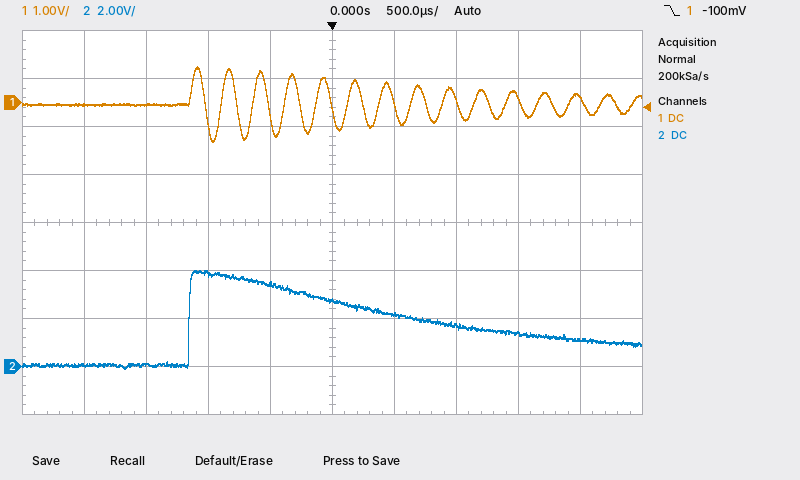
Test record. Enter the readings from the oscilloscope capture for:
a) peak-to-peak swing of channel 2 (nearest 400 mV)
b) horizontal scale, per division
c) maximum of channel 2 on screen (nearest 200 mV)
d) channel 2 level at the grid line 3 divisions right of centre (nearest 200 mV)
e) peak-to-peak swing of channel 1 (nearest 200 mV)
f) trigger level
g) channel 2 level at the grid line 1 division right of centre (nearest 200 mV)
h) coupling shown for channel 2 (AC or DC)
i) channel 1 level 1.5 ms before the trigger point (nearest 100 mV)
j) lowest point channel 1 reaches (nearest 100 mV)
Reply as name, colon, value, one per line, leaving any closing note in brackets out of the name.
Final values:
peak-to-peak swing of channel 2: 4.0 V
horizontal scale, per division: 500 µs
maximum of channel 2 on screen: 4.0 V
channel 2 level at the grid line 3 divisions right of centre: 1.4 V
peak-to-peak swing of channel 1: 1.6 V
trigger level: -100 mV
channel 2 level at the grid line 1 division right of centre: 2.2 V
coupling shown for channel 2: DC
channel 1 level 1.5 ms before the trigger point: 0.0 V
lowest point channel 1 reaches: -800 mV
